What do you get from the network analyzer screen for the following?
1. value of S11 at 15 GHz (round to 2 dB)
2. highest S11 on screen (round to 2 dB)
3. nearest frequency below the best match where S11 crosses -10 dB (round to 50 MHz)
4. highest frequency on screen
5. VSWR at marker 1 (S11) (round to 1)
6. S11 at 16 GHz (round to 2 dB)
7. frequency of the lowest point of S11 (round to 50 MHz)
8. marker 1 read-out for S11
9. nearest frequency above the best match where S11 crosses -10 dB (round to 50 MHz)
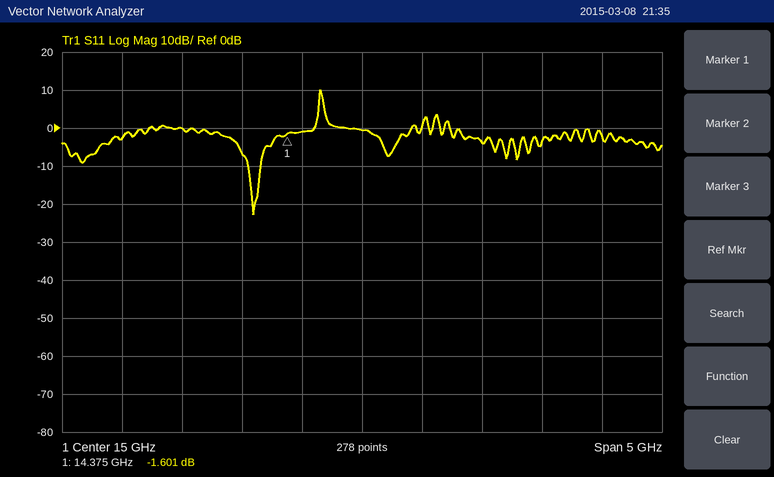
0 dB
10 dB
14.05 GHz
17.5 GHz
11
-4 dB
14.10 GHz
-1.601 dB
14.15 GHz
